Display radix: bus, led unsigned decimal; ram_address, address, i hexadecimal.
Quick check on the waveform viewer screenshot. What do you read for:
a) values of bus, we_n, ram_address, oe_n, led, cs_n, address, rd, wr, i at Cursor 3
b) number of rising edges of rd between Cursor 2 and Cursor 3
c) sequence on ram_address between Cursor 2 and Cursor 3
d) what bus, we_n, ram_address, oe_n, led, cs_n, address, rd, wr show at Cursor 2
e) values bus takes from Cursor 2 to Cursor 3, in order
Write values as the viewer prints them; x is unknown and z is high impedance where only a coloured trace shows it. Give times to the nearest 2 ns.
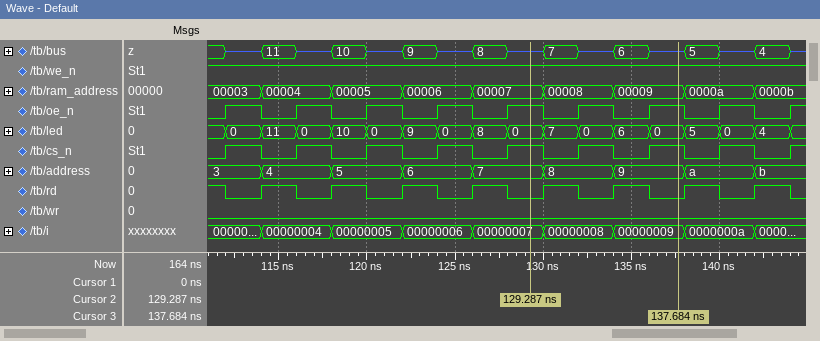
bus=z, we_n=1, ram_address=00009, oe_n=1, led=0, cs_n=1, address=9, rd=0, wr=0, i=00000009
2
00007, 00008, 00009
bus=z, we_n=1, ram_address=00007, oe_n=1, led=0, cs_n=1, address=7, rd=0, wr=0
z, 7, z, 6, z
